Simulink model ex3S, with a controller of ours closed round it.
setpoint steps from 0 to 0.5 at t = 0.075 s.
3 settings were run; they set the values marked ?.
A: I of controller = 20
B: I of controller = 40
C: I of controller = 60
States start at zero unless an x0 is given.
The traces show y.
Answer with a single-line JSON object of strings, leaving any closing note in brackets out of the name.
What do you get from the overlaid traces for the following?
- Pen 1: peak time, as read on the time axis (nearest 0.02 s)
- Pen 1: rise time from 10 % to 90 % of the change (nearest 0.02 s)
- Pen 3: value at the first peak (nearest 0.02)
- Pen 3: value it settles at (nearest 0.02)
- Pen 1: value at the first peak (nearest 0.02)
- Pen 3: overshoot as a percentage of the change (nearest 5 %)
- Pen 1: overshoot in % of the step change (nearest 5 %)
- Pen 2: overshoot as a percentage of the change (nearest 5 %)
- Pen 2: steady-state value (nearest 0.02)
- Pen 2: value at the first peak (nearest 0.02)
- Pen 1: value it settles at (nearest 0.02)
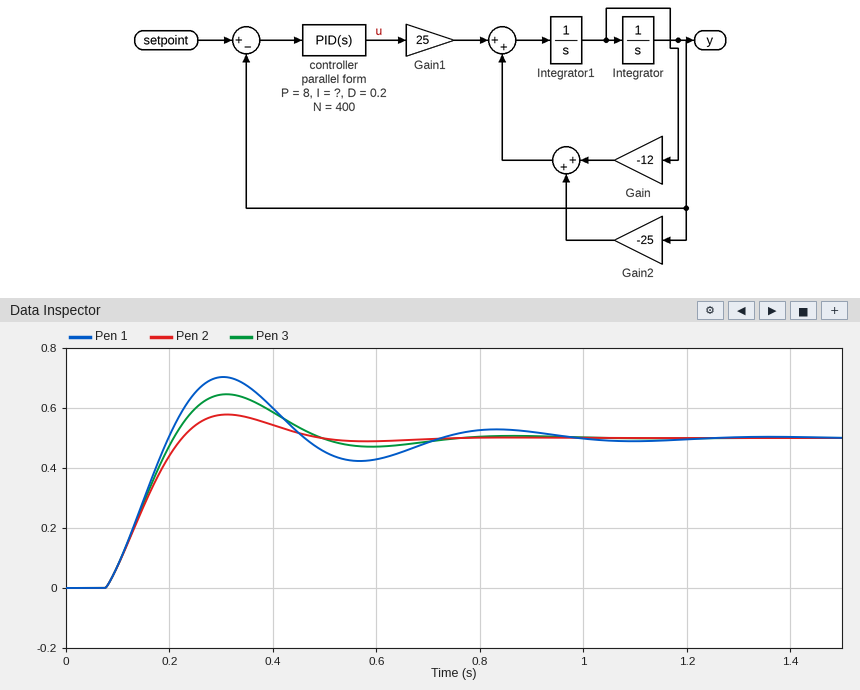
{"Pen 1: peak time, as read on the time axis": "0.30 s", "Pen 1: rise time from 10 % to 90 % of the change": "0.10 s", "Pen 3: value at the first peak": "0.64", "Pen 3: value it settles at": "0.50", "Pen 1: value at the first peak": "0.70", "Pen 3: overshoot as a percentage of the change": "30 %", "Pen 1: overshoot in % of the step change": "40 %", "Pen 2: overshoot as a percentage of the change": "15 %", "Pen 2: steady-state value": "0.50", "Pen 2: value at the first peak": "0.58", "Pen 1: value it settles at": "0.50"}
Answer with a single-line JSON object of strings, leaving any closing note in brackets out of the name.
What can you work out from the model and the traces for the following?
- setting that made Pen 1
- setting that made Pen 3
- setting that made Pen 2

{"setting that made Pen 1": "C", "setting that made Pen 3": "B", "setting that made Pen 2": "A"}
